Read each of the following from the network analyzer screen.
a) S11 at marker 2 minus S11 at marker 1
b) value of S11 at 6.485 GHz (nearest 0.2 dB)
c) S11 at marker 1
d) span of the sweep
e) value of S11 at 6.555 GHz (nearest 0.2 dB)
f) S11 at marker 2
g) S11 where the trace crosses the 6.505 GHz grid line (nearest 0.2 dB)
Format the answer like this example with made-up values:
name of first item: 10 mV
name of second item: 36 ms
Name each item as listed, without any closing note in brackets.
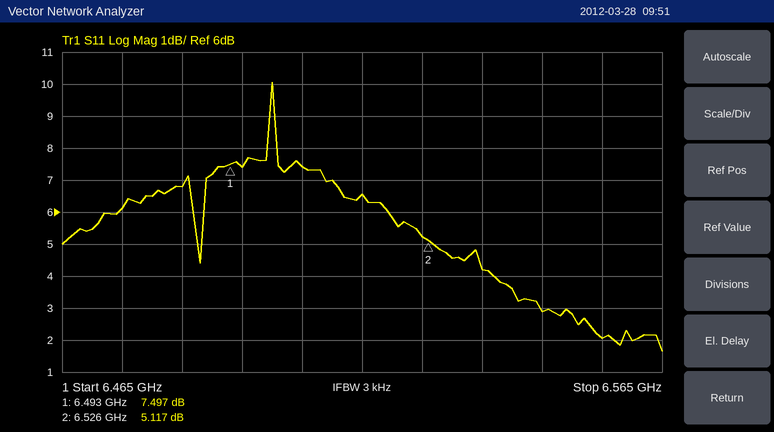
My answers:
S11 at marker 2 minus S11 at marker 1: -2.380 dB
value of S11 at 6.485 GHz: 6.8 dB
S11 at marker 1: 7.497 dB
span of the sweep: 100 MHz
value of S11 at 6.555 GHz: 2.0 dB
S11 at marker 2: 5.117 dB
S11 where the trace crosses the 6.505 GHz grid line: 7.4 dB
